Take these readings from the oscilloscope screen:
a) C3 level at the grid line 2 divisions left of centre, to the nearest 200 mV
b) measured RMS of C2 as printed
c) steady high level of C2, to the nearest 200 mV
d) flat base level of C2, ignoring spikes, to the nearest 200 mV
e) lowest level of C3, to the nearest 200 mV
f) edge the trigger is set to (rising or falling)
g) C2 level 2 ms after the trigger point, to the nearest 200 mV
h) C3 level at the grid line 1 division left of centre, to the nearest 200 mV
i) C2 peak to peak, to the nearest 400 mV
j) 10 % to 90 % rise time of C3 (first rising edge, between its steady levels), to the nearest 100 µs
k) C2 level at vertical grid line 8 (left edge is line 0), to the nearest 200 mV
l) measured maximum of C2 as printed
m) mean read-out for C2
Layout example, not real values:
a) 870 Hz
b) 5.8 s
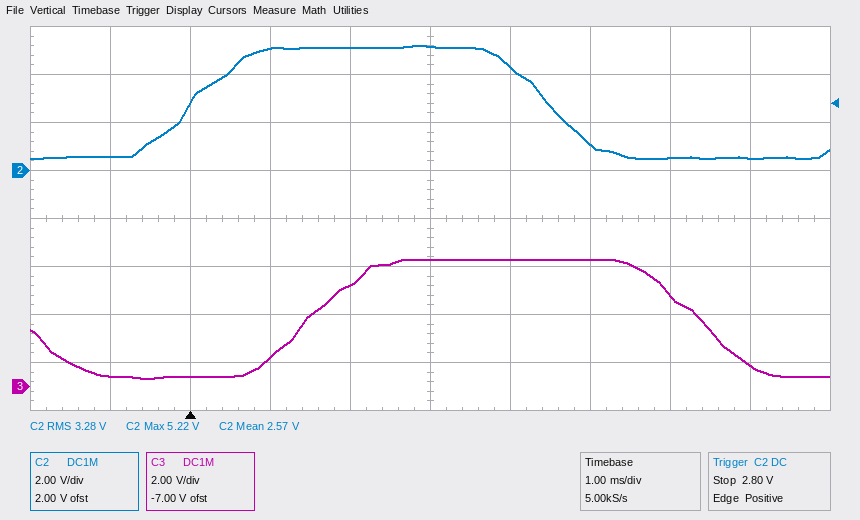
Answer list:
a) 1.2 V
b) 3.28 V
c) 5.2 V
d) 600 mV
e) 400 mV
f) rising
g) 5.2 V
h) 4.2 V
i) 4.8 V
j) 1.3 ms
k) 600 mV
l) 5.22 V
m) 2.57 V
